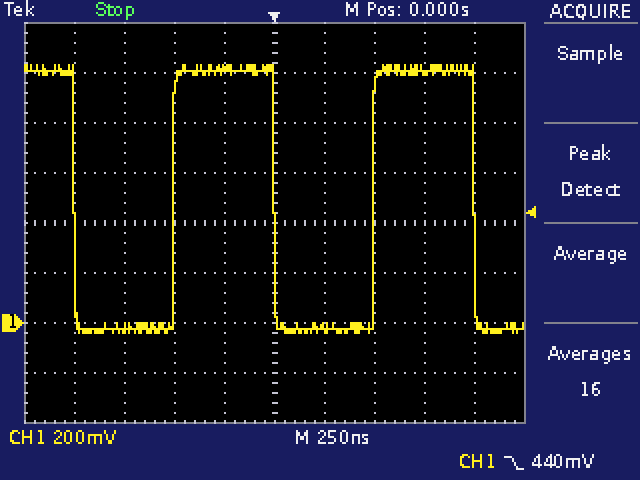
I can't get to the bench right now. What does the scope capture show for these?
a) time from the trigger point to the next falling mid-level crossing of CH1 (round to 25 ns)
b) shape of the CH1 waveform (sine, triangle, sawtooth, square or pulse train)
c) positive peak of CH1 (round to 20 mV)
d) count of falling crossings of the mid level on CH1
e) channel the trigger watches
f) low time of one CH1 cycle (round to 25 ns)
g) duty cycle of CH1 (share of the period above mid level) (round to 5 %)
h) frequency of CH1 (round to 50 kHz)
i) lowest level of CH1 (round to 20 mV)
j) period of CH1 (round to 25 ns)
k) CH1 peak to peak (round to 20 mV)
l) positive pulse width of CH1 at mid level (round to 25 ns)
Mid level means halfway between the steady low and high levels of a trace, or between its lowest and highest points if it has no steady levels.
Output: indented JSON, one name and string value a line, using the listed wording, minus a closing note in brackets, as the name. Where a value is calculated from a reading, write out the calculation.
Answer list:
{
  "time from the trigger point to the next falling mid-level crossing of CH1": "1.000 µs",
  "shape of the CH1 waveform": "square",
  "positive peak of CH1": "1.04 V",
  "count of falling crossings of the mid level on CH1": "3",
  "channel the trigger watches": "CH1",
  "low time of one CH1 cycle": "500 ns",
  "duty cycle of CH1 (share of the period above mid level)": "500 ns / 1.000 µs ≈ 50 %",
  "frequency of CH1": "1 / 1.000 µs ≈ 1.00 MHz",
  "lowest level of CH1": "-40 mV",
  "period of CH1": "1.000 µs",
  "CH1 peak to peak": "1.04 V − (-40 mV) = 1.08 V",
  "positive pulse width of CH1 at mid level": "500 ns"
}
